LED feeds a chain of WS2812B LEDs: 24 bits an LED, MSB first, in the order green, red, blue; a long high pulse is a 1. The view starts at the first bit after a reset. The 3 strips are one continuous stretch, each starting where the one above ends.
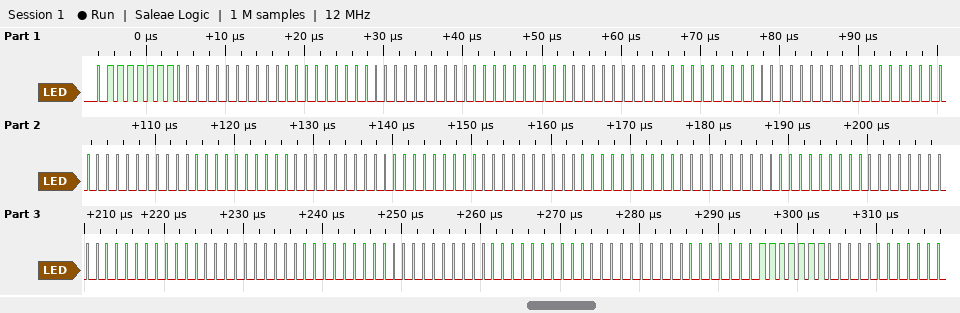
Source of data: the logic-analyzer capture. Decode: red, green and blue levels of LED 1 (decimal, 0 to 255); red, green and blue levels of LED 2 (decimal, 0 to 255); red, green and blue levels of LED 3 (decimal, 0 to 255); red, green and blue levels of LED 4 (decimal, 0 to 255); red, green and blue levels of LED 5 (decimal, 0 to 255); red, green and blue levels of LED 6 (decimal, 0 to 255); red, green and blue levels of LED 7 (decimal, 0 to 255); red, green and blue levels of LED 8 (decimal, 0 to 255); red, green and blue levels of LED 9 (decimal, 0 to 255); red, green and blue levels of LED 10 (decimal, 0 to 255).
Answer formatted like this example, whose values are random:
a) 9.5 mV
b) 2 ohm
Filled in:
a) 0, 127, 0
b) 0, 0, 0
c) 0, 0, 0
d) 0, 0, 0
e) 0, 0, 0
f) 0, 0, 0
g) 0, 0, 0
h) 0, 0, 0
i) 0, 0, 0
j) 0, 0, 0
